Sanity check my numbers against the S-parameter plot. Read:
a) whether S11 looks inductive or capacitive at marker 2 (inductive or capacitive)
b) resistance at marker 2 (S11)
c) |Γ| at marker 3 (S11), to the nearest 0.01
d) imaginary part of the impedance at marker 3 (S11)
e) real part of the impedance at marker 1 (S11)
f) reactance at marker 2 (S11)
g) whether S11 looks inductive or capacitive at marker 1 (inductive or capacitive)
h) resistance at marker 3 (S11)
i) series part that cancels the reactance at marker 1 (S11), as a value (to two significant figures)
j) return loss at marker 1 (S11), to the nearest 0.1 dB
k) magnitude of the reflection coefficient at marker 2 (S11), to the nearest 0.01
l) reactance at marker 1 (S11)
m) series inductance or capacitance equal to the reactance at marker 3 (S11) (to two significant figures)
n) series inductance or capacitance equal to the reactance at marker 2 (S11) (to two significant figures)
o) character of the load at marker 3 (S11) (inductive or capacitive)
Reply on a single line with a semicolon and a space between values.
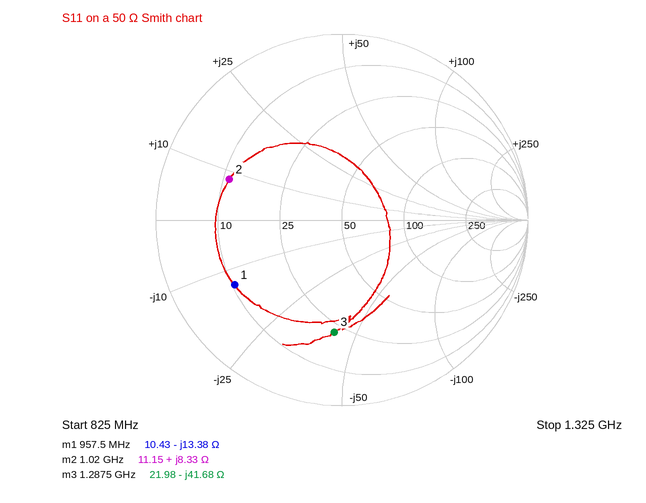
inductive; 11.15 Ω; 0.60; -41.68 Ω; 10.43 Ω; +8.33 Ω; capacitive; 21.98 Ω; 2.2 nH; 3.4 dB; 0.64; -13.38 Ω; 3.0 pF; 1.3 nH; capacitive
